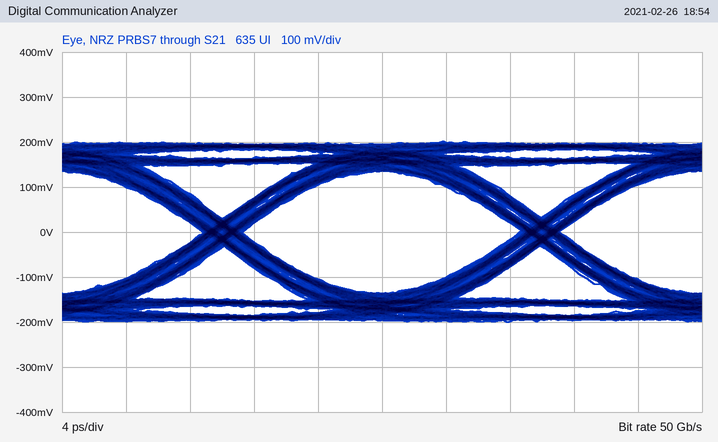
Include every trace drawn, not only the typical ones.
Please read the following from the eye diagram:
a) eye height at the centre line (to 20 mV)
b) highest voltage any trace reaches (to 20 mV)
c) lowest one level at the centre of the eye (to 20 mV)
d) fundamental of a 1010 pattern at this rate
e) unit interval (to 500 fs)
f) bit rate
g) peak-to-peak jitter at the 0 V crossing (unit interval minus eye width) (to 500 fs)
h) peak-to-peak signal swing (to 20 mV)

280 mV
200 mV
140 mV
25 GHz
20.0 ps
50 Gb/s
2.5 ps
400 mV
